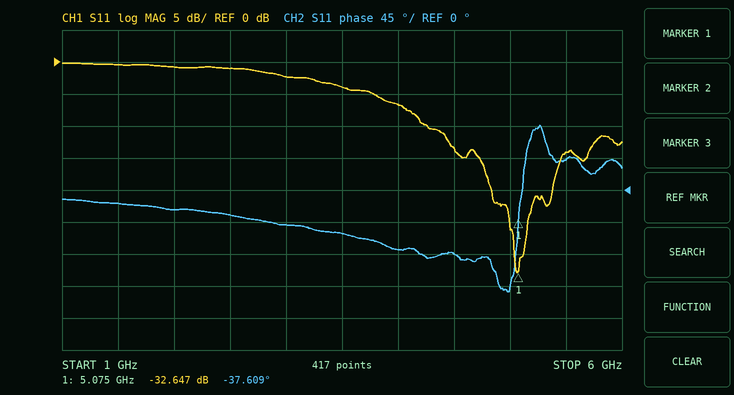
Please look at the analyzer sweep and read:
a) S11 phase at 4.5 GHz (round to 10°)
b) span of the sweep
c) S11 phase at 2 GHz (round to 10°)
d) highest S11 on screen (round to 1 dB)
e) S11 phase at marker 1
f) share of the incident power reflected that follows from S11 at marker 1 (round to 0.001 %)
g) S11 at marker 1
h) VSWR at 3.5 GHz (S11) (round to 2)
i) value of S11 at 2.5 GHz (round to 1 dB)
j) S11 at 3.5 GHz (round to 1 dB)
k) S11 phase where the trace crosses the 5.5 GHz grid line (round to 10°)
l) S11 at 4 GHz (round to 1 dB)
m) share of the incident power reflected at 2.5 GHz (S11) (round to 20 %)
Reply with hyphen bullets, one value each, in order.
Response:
- -90°
- 5 GHz
- -30°
- 0 dB
- -37.609°
- 0.054 %
- -32.647 dB
- 4
- -1 dB
- -4 dB
- 40°
- -7 dB
- 80 %
